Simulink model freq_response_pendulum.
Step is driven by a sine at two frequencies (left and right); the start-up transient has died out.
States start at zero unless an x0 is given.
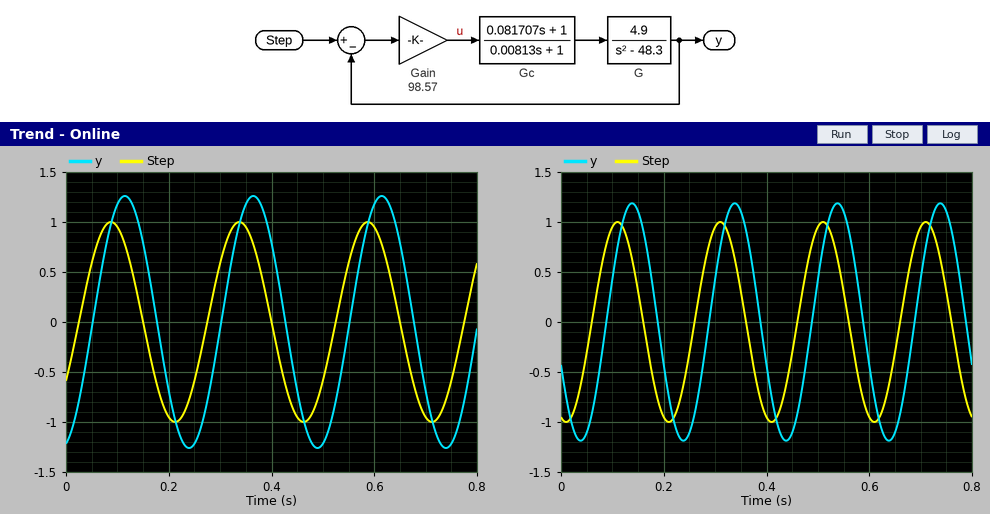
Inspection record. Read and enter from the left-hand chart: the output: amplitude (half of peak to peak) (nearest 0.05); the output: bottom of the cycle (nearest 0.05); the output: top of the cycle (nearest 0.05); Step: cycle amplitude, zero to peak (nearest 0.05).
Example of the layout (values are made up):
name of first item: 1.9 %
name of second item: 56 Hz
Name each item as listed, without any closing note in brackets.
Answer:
the output: amplitude (half of peak to peak): 1.25
the output: bottom of the cycle: -1.25
the output: top of the cycle: 1.25
Step: cycle amplitude, zero to peak: 1.00
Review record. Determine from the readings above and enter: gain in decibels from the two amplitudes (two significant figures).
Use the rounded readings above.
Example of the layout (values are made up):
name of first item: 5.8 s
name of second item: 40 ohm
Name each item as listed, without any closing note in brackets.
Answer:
gain in decibels from the two amplitudes: 1.9 dB
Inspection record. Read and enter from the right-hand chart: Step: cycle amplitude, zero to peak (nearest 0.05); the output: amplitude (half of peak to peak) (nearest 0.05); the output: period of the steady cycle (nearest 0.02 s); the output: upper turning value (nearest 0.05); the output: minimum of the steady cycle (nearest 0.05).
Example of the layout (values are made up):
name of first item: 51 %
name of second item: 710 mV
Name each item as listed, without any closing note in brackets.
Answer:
Step: cycle amplitude, zero to peak: 1.00
the output: amplitude (half of peak to peak): 1.20
the output: period of the steady cycle: 0.20 s
the output: upper turning value: 1.20
the output: minimum of the steady cycle: -1.20
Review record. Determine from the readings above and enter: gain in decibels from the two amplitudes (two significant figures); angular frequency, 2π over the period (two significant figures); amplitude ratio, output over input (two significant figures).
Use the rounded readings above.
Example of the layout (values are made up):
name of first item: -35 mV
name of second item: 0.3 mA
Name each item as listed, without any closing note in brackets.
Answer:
gain in decibels from the two amplitudes: 1.6 dB
angular frequency, 2π over the period: 31 rad/s
amplitude ratio, output over input: 1.2
